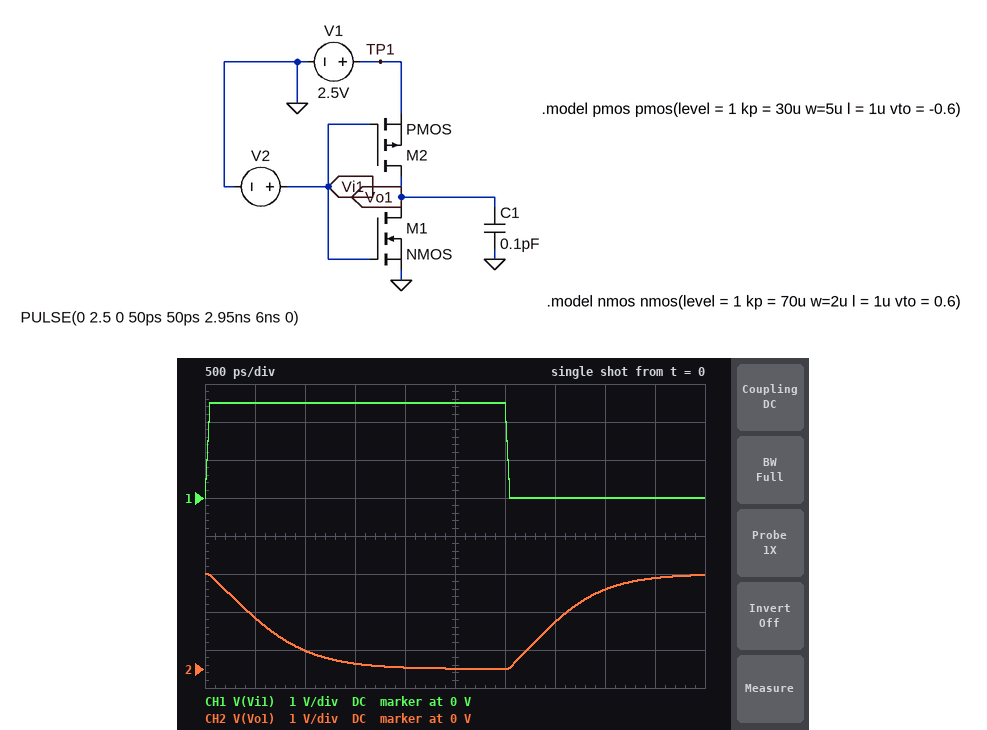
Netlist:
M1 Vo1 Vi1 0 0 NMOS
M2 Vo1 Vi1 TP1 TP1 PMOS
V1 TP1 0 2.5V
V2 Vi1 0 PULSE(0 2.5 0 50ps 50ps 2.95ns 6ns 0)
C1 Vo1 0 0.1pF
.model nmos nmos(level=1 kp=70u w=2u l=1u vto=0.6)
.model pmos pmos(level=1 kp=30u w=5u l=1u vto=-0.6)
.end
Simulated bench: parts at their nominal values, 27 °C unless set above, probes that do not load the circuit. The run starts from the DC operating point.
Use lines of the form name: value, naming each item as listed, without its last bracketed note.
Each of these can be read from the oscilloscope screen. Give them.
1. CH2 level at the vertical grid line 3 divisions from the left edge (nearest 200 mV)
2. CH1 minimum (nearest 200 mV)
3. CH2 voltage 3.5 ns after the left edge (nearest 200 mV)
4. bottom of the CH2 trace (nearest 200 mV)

CH2 level at the vertical grid line 3 divisions from the left edge: 200 mV
CH1 minimum: 0 V
CH2 voltage 3.5 ns after the left edge: 1.2 V
bottom of the CH2 trace: 0 V
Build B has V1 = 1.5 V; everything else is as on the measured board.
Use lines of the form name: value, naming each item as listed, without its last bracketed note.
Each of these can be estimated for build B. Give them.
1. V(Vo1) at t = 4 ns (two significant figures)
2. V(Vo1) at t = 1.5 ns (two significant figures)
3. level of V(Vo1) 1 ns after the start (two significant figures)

V(Vo1) at t = 4 ns: 580 mV
V(Vo1) at t = 1.5 ns: 50 mV
level of V(Vo1) 1 ns after the start: 180 mV
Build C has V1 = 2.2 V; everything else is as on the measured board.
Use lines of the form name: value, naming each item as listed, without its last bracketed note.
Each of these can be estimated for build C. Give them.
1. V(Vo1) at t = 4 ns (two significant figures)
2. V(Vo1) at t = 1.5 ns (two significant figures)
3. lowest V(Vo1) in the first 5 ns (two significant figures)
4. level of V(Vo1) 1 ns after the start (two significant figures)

V(Vo1) at t = 4 ns: 1.6 V
V(Vo1) at t = 1.5 ns: 100 mV
lowest V(Vo1) in the first 5 ns: 1.9 mV
level of V(Vo1) 1 ns after the start: 360 mV
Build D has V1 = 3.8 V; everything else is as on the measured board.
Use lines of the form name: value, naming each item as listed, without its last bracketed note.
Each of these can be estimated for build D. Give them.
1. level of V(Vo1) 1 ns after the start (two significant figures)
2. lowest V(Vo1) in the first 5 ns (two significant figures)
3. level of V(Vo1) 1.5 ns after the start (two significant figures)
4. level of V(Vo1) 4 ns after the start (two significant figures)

level of V(Vo1) 1 ns after the start: 1.7 V
lowest V(Vo1) in the first 5 ns: 160 mV
level of V(Vo1) 1.5 ns after the start: 800 mV
level of V(Vo1) 4 ns after the start: 3.7 V
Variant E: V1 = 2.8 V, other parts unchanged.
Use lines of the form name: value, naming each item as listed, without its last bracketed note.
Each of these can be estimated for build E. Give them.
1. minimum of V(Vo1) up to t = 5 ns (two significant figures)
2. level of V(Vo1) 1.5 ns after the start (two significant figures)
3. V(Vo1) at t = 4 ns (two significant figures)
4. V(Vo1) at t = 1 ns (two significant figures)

minimum of V(Vo1) up to t = 5 ns: 3.6 mV
level of V(Vo1) 1.5 ns after the start: 190 mV
V(Vo1) at t = 4 ns: 2.5 V
V(Vo1) at t = 1 ns: 630 mV
